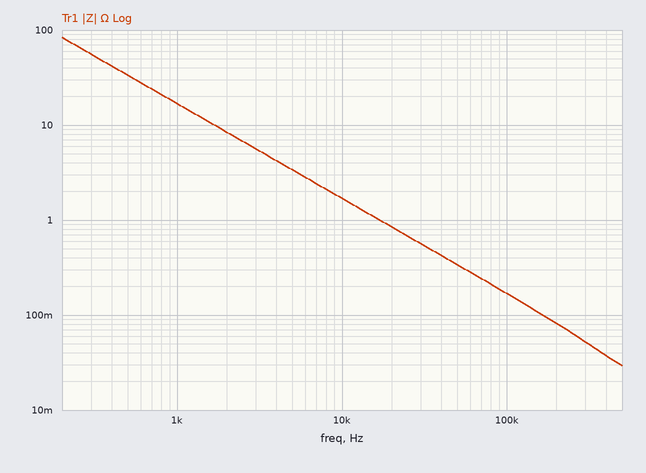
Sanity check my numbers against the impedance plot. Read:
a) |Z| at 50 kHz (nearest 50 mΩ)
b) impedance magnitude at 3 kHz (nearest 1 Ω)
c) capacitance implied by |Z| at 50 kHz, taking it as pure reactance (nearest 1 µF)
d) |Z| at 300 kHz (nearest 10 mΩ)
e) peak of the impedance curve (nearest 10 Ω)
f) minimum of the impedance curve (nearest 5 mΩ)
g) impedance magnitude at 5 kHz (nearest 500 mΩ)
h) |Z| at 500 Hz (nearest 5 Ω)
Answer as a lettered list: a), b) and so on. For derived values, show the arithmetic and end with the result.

a) 350 mΩ
b) 6 Ω
c) C = 1/(2π × 50 kHz × 350 mΩ) ≈ 9 µF
d) 50 mΩ
e) 80 Ω
f) 30 mΩ
g) 3.5 Ω
h) 35 Ω
